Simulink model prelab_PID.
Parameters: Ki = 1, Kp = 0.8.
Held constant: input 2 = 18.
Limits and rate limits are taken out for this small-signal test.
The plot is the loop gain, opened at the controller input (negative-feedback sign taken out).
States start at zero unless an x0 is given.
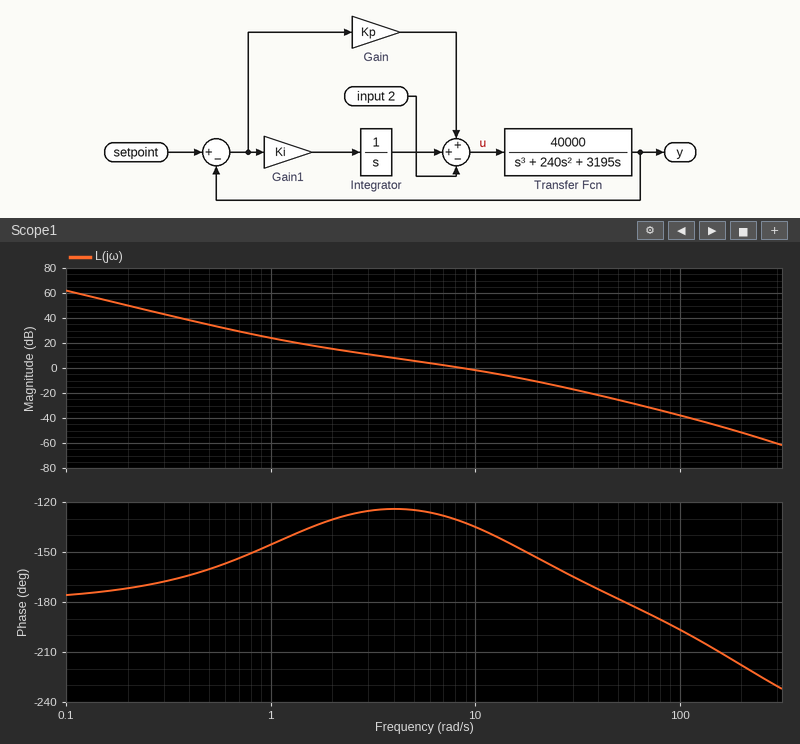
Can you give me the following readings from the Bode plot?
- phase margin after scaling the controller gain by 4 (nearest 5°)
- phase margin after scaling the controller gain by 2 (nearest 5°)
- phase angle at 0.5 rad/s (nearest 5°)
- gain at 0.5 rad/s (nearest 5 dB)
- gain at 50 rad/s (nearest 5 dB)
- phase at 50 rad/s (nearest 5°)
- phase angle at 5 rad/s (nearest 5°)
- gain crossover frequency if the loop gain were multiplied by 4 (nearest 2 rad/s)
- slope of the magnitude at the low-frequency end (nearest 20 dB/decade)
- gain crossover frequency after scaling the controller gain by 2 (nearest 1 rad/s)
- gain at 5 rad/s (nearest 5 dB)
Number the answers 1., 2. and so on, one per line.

1. 25°
2. 35°
3. -160°
4. 35 dB
5. -25 dB
6. -180°
7. -125°
8. 22 rad/s
9. -40 dB/decade
10. 14 rad/s
11. 5 dB
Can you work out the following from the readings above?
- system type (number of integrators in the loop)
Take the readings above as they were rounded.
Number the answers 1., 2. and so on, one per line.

1. 2
